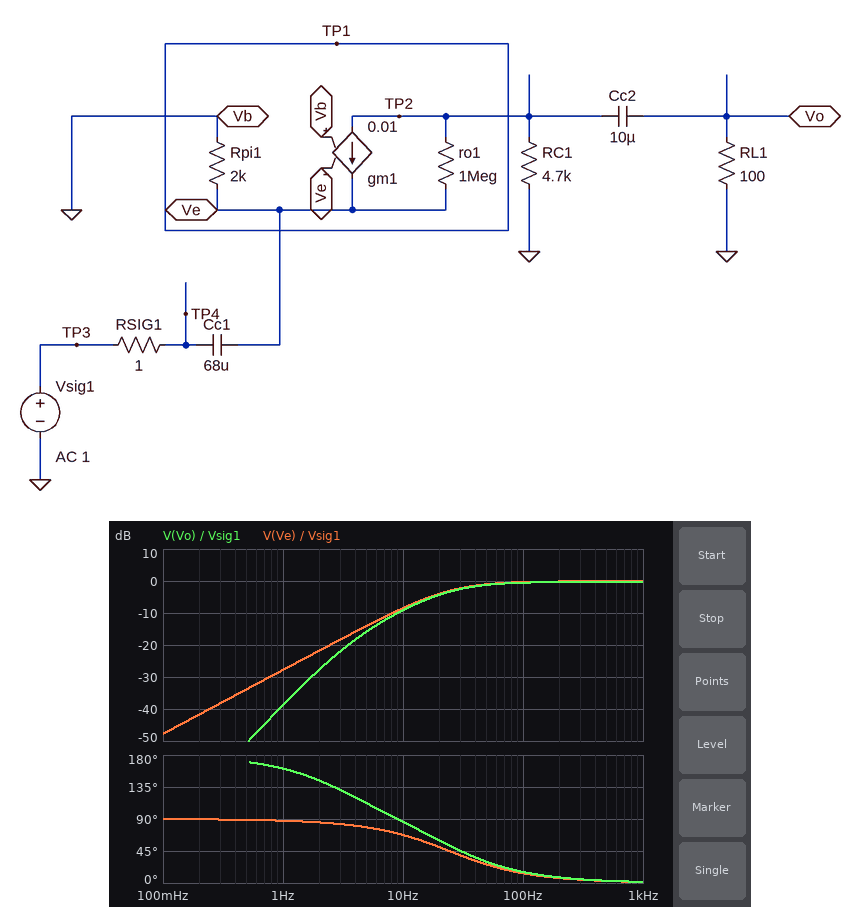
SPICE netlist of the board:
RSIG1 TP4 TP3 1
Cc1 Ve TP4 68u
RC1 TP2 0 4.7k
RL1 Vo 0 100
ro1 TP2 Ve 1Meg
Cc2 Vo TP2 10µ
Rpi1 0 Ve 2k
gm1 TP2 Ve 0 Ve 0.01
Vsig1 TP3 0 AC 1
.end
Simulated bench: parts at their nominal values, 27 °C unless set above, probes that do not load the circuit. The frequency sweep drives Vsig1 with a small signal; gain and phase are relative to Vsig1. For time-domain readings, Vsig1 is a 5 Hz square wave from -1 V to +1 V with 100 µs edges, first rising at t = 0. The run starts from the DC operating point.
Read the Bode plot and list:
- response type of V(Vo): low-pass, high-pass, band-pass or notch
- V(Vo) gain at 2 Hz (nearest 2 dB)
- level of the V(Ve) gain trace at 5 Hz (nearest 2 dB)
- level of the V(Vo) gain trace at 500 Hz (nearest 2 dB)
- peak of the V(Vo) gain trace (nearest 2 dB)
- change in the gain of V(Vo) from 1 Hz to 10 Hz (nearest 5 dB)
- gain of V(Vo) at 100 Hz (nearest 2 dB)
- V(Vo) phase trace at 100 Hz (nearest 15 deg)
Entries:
high-pass
-28 dB
-14 dB
0 dB
0 dB
30 dB
0 dB
15 deg
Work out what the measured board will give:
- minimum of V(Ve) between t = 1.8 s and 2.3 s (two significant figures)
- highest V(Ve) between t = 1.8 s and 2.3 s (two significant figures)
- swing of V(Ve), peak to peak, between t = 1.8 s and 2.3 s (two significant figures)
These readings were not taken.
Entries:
-2.0 V
2.0 V
3.9 V
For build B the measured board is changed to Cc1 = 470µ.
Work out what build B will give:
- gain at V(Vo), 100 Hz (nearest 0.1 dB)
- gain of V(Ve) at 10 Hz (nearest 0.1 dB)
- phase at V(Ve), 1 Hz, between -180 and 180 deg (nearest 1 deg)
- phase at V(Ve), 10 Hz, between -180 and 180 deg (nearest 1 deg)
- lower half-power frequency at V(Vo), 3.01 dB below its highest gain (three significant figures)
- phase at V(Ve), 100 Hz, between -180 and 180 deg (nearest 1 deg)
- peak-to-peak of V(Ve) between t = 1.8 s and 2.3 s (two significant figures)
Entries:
-0.3 dB
-0.6 dB
74 deg
19 deg
5.33 Hz
2 deg
3.6 V
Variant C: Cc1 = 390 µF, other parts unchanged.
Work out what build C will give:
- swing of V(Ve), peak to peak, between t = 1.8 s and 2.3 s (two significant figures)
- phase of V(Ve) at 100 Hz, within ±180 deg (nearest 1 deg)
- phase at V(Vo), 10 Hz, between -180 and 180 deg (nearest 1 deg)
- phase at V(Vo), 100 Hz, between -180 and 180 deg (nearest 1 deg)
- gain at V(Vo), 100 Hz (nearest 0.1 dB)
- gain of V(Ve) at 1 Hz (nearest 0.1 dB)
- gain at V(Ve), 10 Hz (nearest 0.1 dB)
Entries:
3.7 V
2 deg
41 deg
4 deg
-0.3 dB
-12.8 dB
-0.8 dB
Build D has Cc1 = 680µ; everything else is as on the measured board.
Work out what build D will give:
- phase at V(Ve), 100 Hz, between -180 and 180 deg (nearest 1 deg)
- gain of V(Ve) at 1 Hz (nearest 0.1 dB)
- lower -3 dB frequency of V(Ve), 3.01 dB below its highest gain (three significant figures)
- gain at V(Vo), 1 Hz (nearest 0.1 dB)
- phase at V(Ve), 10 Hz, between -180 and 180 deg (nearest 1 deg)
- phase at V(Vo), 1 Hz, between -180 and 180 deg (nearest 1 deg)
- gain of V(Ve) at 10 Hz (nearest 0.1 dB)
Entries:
1 deg
-8.5 dB
2.43 Hz
-19.5 dB
14 deg
141 deg
-0.3 dB
